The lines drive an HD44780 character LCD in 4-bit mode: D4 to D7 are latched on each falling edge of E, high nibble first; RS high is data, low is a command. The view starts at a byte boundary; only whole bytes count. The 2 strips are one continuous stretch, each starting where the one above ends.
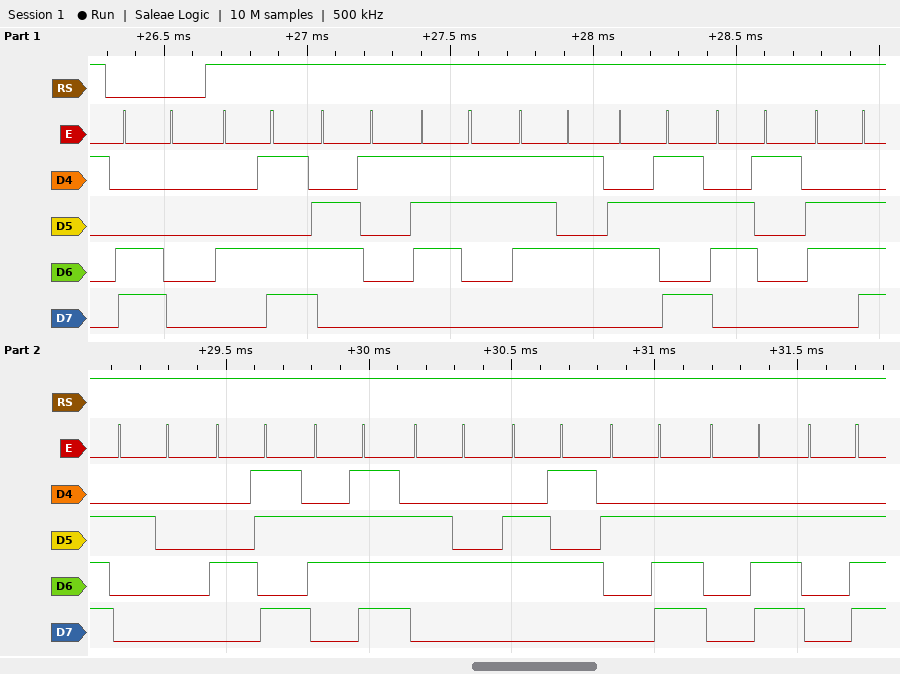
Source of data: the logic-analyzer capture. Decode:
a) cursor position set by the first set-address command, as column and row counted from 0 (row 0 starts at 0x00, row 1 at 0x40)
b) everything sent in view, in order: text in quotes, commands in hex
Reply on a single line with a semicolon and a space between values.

column 0, row 1; 0xC0 "Masukan Kode..."
